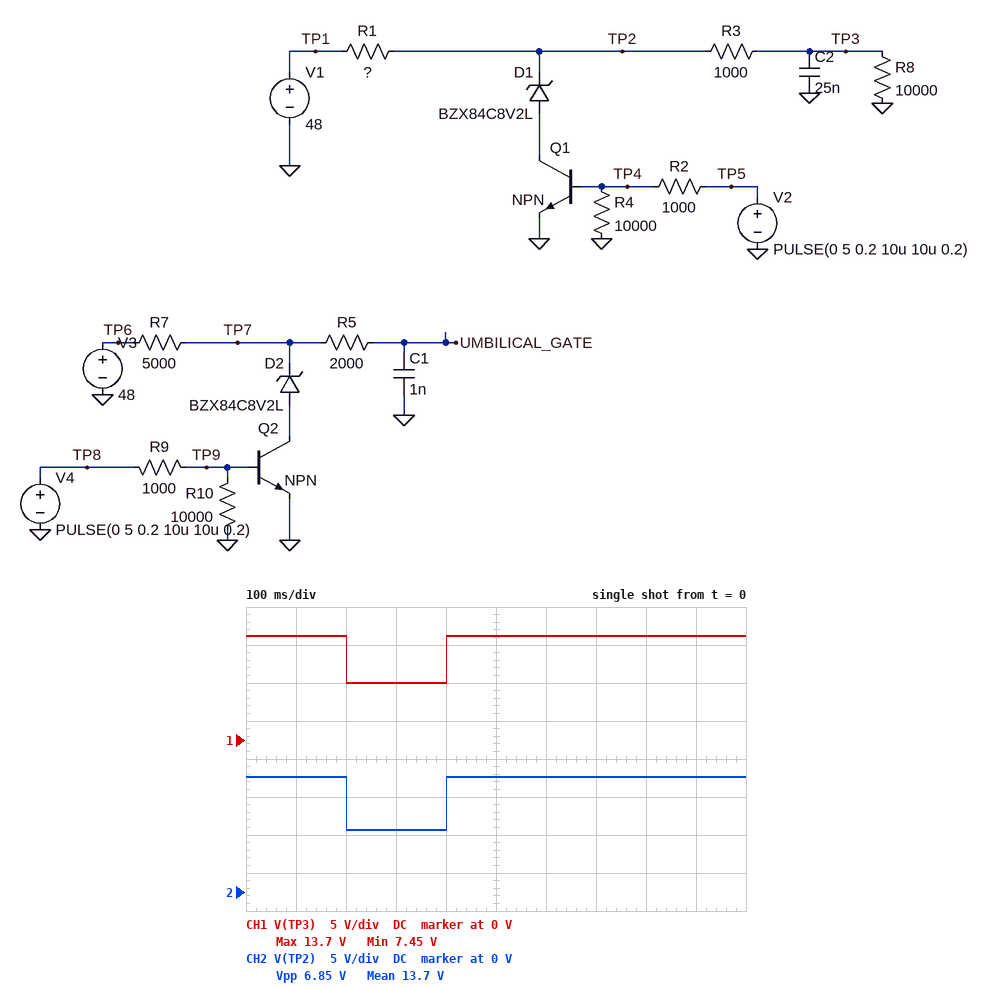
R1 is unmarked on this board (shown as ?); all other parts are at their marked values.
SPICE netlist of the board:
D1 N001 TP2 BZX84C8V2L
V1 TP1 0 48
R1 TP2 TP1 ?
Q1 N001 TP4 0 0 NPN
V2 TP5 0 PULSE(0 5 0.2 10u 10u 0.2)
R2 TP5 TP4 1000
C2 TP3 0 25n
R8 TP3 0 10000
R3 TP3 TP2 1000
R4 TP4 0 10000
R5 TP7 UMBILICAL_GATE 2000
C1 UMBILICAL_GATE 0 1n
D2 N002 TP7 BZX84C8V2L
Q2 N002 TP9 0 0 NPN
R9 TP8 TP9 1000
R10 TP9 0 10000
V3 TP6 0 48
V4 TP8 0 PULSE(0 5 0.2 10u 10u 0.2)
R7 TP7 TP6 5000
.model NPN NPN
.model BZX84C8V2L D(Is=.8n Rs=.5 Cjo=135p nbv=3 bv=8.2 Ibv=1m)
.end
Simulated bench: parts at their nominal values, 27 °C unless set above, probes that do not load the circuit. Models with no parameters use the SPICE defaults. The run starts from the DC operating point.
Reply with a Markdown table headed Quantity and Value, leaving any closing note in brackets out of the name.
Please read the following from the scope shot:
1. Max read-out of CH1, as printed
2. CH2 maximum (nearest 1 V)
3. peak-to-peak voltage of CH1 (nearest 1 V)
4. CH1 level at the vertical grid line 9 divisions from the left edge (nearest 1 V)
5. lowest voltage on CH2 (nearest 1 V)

| Quantity | Value |
|---|---|
| Max read-out of CH1, as printed | 13.7 V |
| CH2 maximum | 15 V |
| peak-to-peak voltage of CH1 | 6 V |
| CH1 level at the vertical grid line 9 divisions from the left edge | 14 V |
| lowest voltage on CH2 | 8 V |
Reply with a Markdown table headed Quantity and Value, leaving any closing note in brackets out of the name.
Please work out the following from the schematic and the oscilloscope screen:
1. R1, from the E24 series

| Quantity | Value |
|---|---|
| R1, from the E24 series | 24 kΩ |
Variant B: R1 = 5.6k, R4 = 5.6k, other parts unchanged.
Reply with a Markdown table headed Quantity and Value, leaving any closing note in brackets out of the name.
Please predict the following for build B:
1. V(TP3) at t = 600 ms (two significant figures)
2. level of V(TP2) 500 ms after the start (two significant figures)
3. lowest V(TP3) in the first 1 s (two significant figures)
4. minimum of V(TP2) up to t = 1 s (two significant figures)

| Quantity | Value |
|---|---|
| V(TP3) at t = 600 ms | 29 V |
| level of V(TP2) 500 ms after the start | 32 V |
| lowest V(TP3) in the first 1 s | 7.6 V |
| minimum of V(TP2) up to t = 1 s | 8.4 V |
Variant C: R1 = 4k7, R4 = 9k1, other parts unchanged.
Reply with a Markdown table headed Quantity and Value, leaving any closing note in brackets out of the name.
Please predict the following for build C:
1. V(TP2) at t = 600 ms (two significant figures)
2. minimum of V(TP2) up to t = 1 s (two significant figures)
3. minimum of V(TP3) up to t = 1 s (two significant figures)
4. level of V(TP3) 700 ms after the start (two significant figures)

| Quantity | Value |
|---|---|
| V(TP2) at t = 600 ms | 34 V |
| minimum of V(TP2) up to t = 1 s | 8.4 V |
| minimum of V(TP3) up to t = 1 s | 7.6 V |
| level of V(TP3) 700 ms after the start | 31 V |
